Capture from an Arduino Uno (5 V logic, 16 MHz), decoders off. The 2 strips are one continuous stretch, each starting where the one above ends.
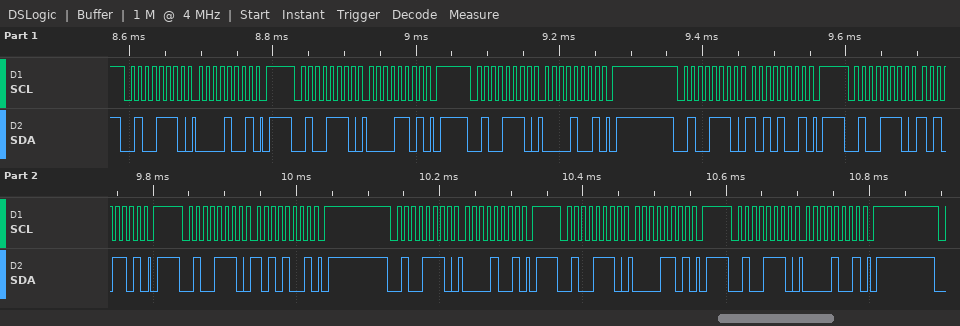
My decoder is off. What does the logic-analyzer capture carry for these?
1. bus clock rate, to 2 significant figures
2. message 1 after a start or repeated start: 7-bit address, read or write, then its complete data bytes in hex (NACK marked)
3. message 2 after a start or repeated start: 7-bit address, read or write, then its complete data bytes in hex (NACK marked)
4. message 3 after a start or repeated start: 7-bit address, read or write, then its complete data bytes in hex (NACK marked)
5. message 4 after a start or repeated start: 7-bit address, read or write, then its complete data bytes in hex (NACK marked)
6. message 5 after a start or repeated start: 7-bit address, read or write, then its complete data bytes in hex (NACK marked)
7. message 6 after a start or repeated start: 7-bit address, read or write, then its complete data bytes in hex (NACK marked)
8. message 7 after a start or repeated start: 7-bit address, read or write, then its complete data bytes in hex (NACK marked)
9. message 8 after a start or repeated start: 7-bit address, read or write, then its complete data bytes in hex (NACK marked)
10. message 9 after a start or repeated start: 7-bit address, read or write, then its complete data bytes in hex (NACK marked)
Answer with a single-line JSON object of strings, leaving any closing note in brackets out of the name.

{"bus clock rate, to 2 significant figures": "100 kHz", "message 1 after a start or repeated start: 7-bit address, read or write, then its complete data bytes in hex": "0x27 write: 09", "message 2 after a start or repeated start: 7-bit address, read or write, then its complete data bytes in hex": "0x27 write: 0D", "message 3 after a start or repeated start: 7-bit address, read or write, then its complete data bytes in hex": "0x27 write: 09", "message 4 after a start or repeated start: 7-bit address, read or write, then its complete data bytes in hex": "0x27 write: A9", "message 5 after a start or repeated start: 7-bit address, read or write, then its complete data bytes in hex": "0x27 write: AD", "message 6 after a start or repeated start: 7-bit address, read or write, then its complete data bytes in hex": "0x27 write: A9", "message 7 after a start or repeated start: 7-bit address, read or write, then its complete data bytes in hex": "0x27 write: 09", "message 8 after a start or repeated start: 7-bit address, read or write, then its complete data bytes in hex": "0x27 write: 0D", "message 9 after a start or repeated start: 7-bit address, read or write, then its complete data bytes in hex": "0x27 write: 09"}
